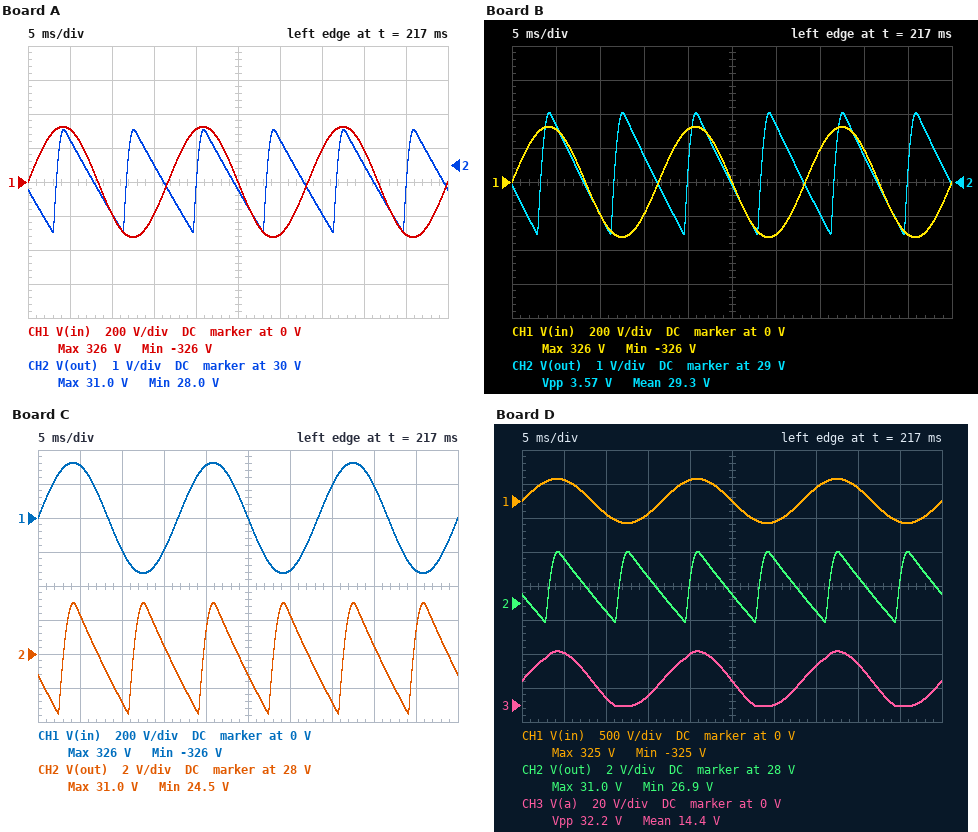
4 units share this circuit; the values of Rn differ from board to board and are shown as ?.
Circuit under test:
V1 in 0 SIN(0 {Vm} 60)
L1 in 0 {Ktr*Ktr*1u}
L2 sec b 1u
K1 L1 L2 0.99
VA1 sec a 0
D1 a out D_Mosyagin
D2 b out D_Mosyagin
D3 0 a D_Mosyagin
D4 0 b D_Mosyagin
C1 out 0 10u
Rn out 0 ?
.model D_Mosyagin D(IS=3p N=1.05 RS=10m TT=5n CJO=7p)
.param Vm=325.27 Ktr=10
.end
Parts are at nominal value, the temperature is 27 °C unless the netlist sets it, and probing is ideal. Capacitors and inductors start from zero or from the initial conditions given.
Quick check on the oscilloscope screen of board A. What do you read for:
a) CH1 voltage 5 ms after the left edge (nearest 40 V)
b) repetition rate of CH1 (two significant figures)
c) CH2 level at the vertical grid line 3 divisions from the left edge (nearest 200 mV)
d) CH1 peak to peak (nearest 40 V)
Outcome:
320 V
60 Hz
30.0 V
640 V
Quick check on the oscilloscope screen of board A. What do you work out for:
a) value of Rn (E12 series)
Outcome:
6.8 kΩ
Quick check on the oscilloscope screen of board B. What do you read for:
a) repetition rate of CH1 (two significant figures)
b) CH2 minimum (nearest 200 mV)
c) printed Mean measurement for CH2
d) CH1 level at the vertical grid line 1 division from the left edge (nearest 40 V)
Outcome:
60 Hz
27.4 V
29.3 V
320 V
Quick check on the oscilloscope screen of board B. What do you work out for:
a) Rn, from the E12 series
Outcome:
5.6 kΩ
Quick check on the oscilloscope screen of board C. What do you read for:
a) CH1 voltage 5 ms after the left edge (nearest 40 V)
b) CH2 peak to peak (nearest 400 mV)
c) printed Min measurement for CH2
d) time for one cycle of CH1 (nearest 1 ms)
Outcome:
320 V
6.4 V
24.5 V
17 ms
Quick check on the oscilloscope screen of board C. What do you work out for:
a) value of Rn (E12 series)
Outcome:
2.7 kΩ
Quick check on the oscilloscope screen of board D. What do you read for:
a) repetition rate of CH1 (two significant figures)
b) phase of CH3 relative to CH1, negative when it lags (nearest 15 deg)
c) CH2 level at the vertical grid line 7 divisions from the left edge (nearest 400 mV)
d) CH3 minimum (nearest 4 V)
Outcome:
60 Hz
0 deg
27.6 V
0 V
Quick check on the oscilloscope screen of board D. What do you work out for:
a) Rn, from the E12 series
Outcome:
4.7 kΩ
